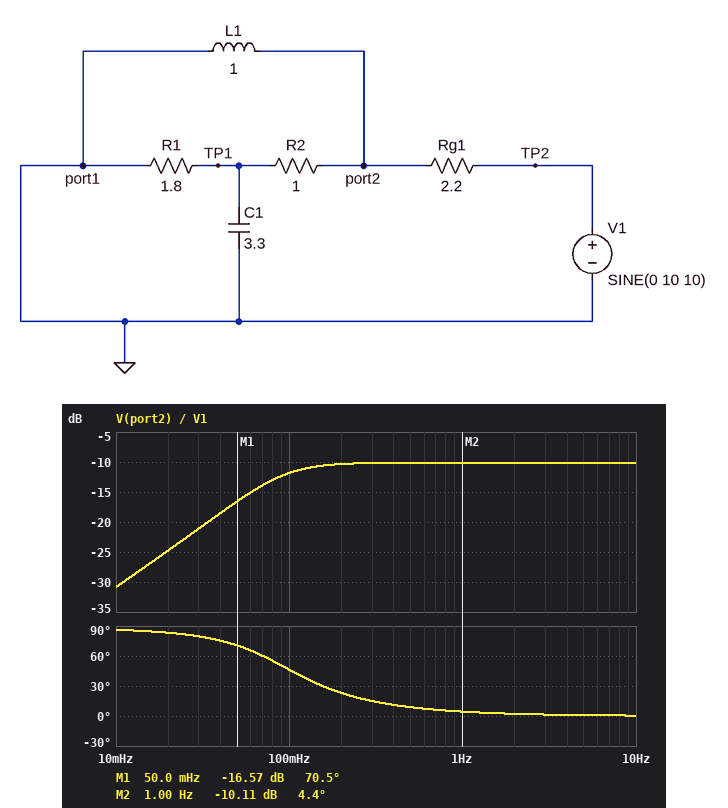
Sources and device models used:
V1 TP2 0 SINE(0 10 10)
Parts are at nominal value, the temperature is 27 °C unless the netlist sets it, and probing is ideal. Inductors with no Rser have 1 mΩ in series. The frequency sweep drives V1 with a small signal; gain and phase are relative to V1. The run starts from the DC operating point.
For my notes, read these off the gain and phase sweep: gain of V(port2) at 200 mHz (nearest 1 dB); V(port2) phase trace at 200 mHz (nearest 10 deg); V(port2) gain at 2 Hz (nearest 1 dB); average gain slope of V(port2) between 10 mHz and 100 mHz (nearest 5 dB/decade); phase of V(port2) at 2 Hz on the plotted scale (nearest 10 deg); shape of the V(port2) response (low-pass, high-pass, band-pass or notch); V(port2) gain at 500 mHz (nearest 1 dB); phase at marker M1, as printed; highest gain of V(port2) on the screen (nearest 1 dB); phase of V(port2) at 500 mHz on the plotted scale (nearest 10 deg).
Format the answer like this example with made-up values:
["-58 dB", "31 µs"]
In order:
["-10 dB", "20 deg", "-10 dB", "20 dB/decade", "0 deg", "high-pass", "-10 dB", "70.5 deg", "-10 dB", "10 deg"]
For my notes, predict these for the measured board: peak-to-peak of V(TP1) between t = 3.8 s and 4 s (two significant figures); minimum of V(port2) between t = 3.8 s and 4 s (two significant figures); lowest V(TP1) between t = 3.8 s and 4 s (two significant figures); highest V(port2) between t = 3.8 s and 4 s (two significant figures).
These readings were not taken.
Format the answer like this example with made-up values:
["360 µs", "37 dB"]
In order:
["30 mV", "-3.1 V", "-18 mV", "3.1 V"]
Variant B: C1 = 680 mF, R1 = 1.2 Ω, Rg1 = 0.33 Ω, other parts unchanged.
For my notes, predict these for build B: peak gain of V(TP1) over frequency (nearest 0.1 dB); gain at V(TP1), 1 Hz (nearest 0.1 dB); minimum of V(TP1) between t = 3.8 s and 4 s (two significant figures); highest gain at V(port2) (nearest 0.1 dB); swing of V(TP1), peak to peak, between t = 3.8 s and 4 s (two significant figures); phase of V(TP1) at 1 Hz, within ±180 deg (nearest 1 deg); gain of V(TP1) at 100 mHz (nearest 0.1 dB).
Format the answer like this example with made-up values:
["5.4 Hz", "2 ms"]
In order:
["-7.4 dB", "-15.6 dB", "-180 mV", "-1.6 dB", "350 mV", "-67 deg", "-7.5 dB"]
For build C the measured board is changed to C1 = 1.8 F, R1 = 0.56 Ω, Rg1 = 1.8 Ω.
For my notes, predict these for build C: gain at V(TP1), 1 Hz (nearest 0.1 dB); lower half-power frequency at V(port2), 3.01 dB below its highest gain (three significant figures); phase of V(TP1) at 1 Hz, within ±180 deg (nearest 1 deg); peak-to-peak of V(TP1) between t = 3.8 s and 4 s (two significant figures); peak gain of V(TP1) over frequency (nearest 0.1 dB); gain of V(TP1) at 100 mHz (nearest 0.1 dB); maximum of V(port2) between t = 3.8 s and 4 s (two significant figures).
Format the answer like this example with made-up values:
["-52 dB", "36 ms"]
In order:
["-30.2 dB", "90.9 mHz", "-73 deg", "63 mV", "-19.3 dB", "-20.4 dB", "3.6 V"]
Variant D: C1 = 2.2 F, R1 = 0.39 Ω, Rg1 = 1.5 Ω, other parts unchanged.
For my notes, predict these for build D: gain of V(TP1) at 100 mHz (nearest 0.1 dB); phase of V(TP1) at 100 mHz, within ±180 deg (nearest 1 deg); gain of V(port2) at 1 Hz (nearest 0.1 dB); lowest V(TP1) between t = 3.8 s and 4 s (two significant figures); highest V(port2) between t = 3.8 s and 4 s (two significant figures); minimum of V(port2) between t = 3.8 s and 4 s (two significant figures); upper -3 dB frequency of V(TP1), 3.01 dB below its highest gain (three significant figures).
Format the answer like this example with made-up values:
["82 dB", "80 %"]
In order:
["-21.5 dB", "25 deg", "-7.9 dB", "-31 mV", "4.0 V", "-4.0 V", "376 mHz"]
